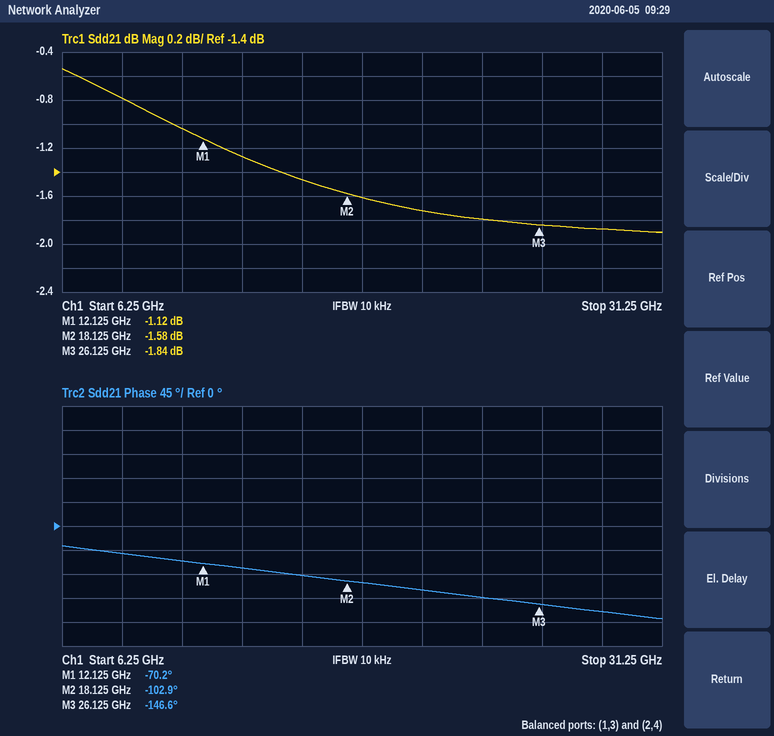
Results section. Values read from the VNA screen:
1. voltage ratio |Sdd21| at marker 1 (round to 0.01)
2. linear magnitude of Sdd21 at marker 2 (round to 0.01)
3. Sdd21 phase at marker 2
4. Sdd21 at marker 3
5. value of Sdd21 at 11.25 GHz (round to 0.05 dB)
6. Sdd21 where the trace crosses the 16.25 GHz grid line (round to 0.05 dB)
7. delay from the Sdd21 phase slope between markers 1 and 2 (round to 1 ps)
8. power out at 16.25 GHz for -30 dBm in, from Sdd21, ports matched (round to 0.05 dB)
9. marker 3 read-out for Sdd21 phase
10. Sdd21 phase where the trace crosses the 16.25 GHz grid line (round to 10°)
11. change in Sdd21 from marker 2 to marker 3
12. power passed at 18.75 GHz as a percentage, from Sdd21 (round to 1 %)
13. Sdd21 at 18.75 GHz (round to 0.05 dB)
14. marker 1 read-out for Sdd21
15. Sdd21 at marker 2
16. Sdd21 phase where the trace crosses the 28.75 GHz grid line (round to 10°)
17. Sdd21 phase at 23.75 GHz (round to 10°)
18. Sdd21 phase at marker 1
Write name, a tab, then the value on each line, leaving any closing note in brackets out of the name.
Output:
voltage ratio |Sdd21| at marker 1	0.88
linear magnitude of Sdd21 at marker 2	0.83
Sdd21 phase at marker 2	-102.9°
Sdd21 at marker 3	-1.84 dB
value of Sdd21 at 11.25 GHz	-1.05 dB
Sdd21 where the trace crosses the 16.25 GHz grid line	-1.45 dB
delay from the Sdd21 phase slope between markers 1 and 2	15 ps
power out at 16.25 GHz for -30 dBm in, from Sdd21, ports matched	-31.45 dBm
marker 3 read-out for Sdd21 phase	-146.6°
Sdd21 phase where the trace crosses the 16.25 GHz grid line	-90°
change in Sdd21 from marker 2 to marker 3	-0.26 dB
power passed at 18.75 GHz as a percentage, from Sdd21	69 %
Sdd21 at 18.75 GHz	-1.60 dB
marker 1 read-out for Sdd21	-1.12 dB
Sdd21 at marker 2	-1.58 dB
Sdd21 phase where the trace crosses the 28.75 GHz grid line	-160°
Sdd21 phase at 23.75 GHz	-130°
Sdd21 phase at marker 1	-70.2°
